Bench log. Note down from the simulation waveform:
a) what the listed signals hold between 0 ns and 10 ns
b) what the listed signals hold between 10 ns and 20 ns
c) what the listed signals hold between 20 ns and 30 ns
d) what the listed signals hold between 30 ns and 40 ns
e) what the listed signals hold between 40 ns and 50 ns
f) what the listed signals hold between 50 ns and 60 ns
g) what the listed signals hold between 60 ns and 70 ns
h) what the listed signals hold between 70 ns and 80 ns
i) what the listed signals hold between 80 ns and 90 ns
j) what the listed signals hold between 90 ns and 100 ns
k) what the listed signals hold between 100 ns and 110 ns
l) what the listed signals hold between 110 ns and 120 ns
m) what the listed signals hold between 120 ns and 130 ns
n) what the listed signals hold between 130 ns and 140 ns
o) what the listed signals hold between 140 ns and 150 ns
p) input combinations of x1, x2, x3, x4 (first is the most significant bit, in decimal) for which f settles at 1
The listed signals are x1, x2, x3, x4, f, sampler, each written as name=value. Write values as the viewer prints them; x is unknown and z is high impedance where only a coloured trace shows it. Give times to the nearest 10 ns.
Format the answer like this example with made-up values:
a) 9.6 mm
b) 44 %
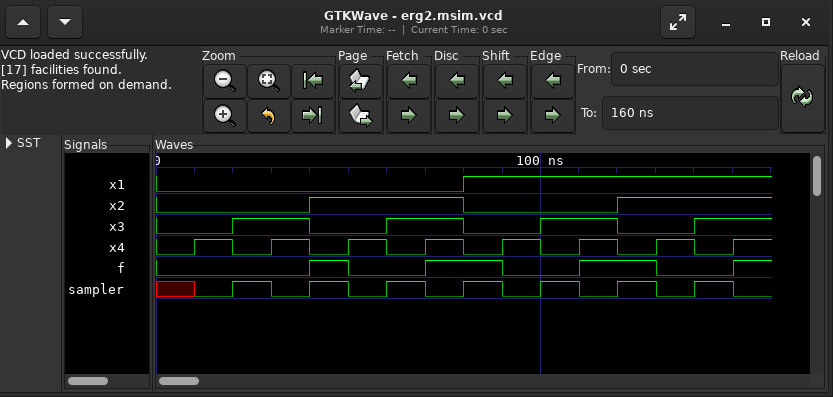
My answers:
a) x1=0, x2=0, x3=0, x4=0, f=0, sampler=x
b) x1=0, x2=0, x3=0, x4=1, f=0, sampler=0
c) x1=0, x2=0, x3=1, x4=0, f=0, sampler=1
d) x1=0, x2=0, x3=1, x4=1, f=0, sampler=0
e) x1=0, x2=1, x3=0, x4=0, f=1, sampler=1
f) x1=0, x2=1, x3=0, x4=1, f=0, sampler=0
g) x1=0, x2=1, x3=1, x4=0, f=0, sampler=1
h) x1=0, x2=1, x3=1, x4=1, f=1, sampler=0
i) x1=1, x2=0, x3=0, x4=0, f=1, sampler=1
j) x1=1, x2=0, x3=0, x4=1, f=0, sampler=0
k) x1=1, x2=0, x3=1, x4=0, f=0, sampler=1
l) x1=1, x2=0, x3=1, x4=1, f=1, sampler=0
m) x1=1, x2=1, x3=0, x4=0, f=1, sampler=1
n) x1=1, x2=1, x3=0, x4=1, f=0, sampler=0
o) x1=1, x2=1, x3=1, x4=0, f=0, sampler=1
p) 4, 7, 8, 11, 12, 15
